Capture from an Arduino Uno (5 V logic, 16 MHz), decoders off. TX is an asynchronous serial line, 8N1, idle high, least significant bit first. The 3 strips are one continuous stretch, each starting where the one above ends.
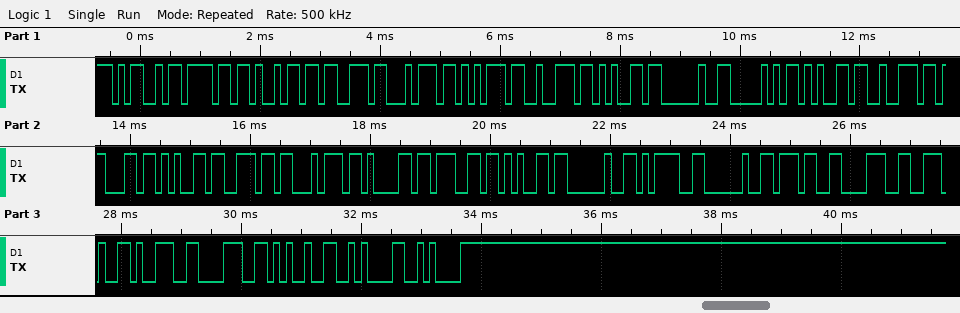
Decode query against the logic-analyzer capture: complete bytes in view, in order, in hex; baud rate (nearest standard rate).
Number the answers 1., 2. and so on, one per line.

1. 4D 6F 69 73 74 75 72 65 20 50 65 72 63 65 6E 74 61 67 65 20 3D 20 37 38 2E 39 38 25 0A 0A
2. 9600 baud
